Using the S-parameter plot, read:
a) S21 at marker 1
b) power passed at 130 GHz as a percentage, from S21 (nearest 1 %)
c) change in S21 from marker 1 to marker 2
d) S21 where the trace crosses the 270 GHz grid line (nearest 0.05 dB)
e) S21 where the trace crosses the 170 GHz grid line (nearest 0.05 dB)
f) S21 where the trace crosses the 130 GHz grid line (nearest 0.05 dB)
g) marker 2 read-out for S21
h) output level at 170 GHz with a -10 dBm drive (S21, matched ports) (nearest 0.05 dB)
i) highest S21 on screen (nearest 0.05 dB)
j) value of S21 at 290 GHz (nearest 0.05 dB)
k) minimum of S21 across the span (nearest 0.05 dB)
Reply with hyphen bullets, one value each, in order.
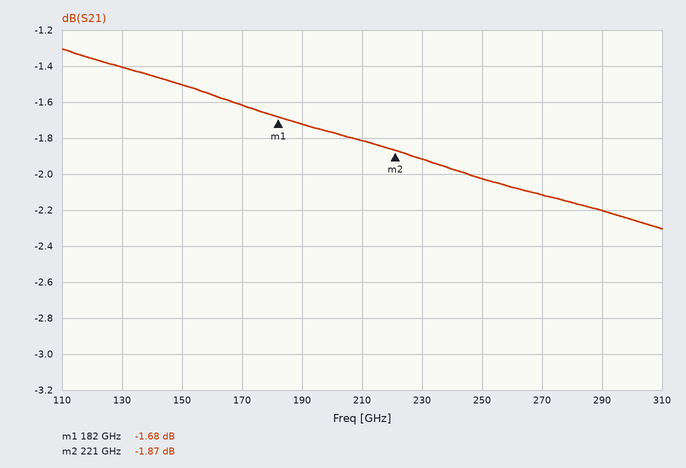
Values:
- -1.68 dB
- 72 %
- -0.19 dB
- -2.10 dB
- -1.60 dB
- -1.40 dB
- -1.87 dB
- -11.60 dBm
- -1.30 dB
- -2.20 dB
- -2.30 dB
